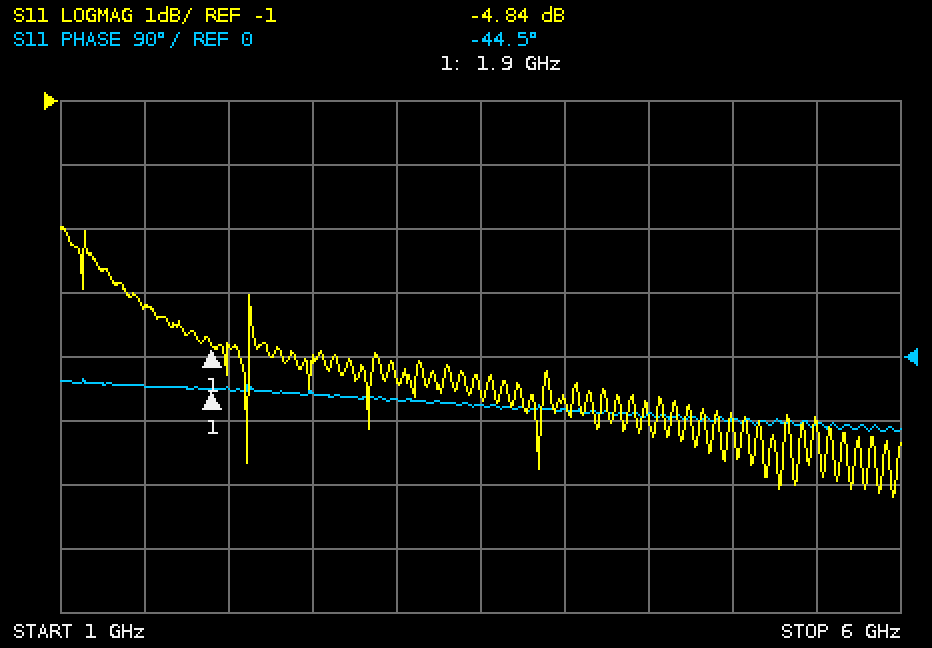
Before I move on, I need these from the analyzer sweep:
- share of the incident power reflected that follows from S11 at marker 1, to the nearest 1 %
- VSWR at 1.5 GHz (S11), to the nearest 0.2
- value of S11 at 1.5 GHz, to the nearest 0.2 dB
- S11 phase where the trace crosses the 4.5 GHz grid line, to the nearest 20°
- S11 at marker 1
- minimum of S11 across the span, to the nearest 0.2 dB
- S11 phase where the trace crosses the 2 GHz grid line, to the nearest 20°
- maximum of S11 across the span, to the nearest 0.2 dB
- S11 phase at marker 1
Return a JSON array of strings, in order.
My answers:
["33 %", "4.2", "-4.2 dB", "-80°", "-4.84 dB", "-7.2 dB", "-40°", "-3.0 dB", "-44.5°"]
